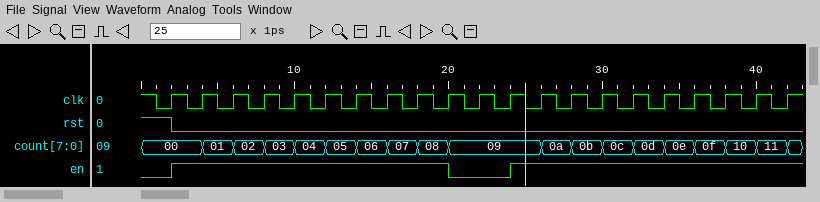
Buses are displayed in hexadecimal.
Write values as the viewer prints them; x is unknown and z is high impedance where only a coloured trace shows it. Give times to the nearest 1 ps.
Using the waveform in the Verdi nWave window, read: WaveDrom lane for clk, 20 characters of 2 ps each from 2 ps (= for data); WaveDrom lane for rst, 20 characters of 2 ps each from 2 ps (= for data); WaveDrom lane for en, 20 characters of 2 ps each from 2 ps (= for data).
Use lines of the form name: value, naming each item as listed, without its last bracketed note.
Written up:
WaveDrom lane for clk, 20 characters of 2 ps each from 2 ps: {name: 'clk', wave: 'p...................'}
WaveDrom lane for rst, 20 characters of 2 ps each from 2 ps: {name: 'rst', wave: '0...................'}
WaveDrom lane for en, 20 characters of 2 ps each from 2 ps: {name: 'en', wave: '1........0.1........'}
